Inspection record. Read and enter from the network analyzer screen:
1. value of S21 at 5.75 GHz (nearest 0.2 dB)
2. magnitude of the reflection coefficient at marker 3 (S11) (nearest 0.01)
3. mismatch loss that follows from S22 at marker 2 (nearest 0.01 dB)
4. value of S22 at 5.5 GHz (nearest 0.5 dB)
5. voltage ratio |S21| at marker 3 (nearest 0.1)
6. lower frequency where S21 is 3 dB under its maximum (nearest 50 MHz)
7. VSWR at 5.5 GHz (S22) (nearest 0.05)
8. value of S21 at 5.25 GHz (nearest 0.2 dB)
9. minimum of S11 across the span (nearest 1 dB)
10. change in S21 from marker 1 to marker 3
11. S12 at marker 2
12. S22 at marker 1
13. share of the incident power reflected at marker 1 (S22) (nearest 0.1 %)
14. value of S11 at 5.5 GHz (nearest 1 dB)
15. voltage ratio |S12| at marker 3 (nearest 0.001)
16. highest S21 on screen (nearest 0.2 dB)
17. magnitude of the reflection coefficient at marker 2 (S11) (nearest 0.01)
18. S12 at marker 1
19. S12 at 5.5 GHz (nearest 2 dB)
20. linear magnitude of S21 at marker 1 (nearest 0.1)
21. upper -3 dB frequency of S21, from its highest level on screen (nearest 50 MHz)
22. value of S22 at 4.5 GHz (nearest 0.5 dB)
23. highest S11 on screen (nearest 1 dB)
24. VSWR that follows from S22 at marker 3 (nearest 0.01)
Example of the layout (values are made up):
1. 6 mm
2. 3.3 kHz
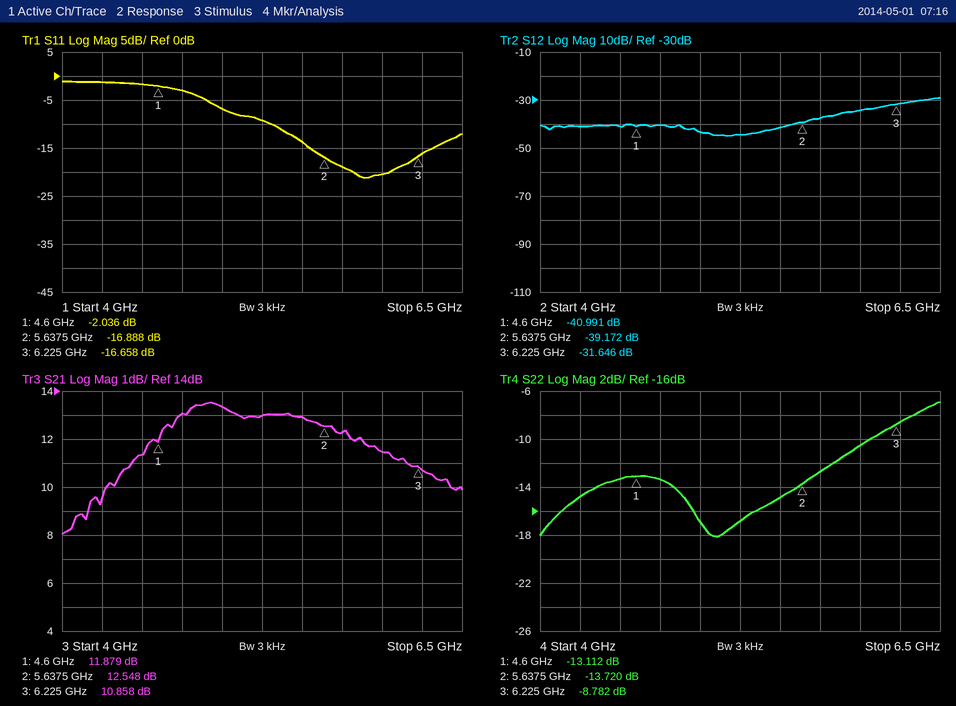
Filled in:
1. 12.2 dB
2. 0.15
3. 0.19 dB
4. -15.0 dB
5. 3.5
6. 4.35 GHz
7. 1.45
8. 13.0 dB
9. -21 dB
10. -1.021 dB
11. -39.172 dB
12. -13.112 dB
13. 4.9 %
14. -14 dB
15. 0.026
16. 13.6 dB
17. 0.14
18. -40.991 dB
19. -42 dB
20. 3.9
21. 6.30 GHz
22. -13.5 dB
23. -1 dB
24. 2.14
